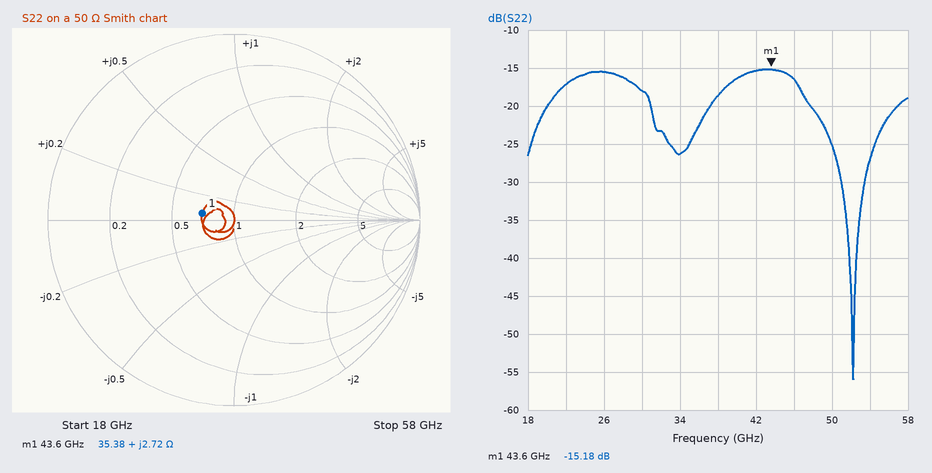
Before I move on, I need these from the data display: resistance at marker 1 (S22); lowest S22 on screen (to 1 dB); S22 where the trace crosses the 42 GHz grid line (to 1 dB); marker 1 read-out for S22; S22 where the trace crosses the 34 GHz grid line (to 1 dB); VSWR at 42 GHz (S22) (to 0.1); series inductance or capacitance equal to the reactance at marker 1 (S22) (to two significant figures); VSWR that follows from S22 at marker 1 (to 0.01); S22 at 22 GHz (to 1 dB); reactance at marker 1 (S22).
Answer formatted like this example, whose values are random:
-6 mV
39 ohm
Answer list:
35.38 Ω
-56 dB
-15 dB
-15.18 dB
-26 dB
1.4
9.9 pH
1.42
-17 dB
+2.72 Ω
